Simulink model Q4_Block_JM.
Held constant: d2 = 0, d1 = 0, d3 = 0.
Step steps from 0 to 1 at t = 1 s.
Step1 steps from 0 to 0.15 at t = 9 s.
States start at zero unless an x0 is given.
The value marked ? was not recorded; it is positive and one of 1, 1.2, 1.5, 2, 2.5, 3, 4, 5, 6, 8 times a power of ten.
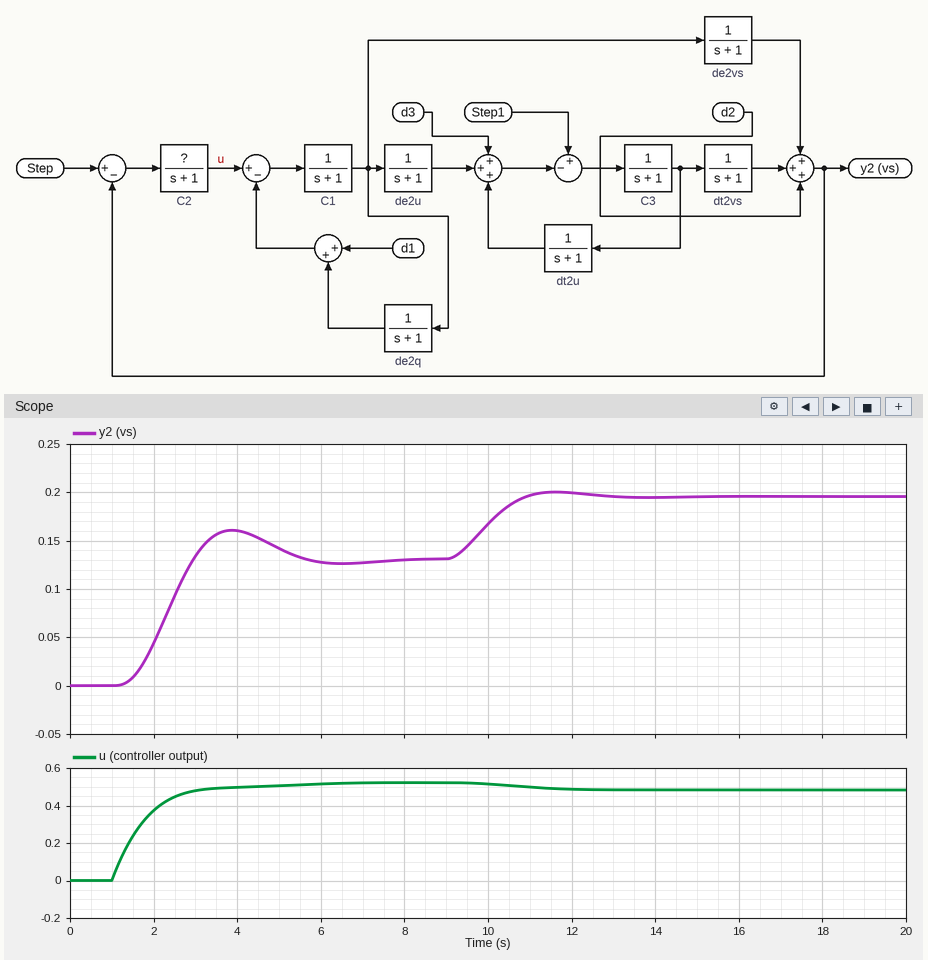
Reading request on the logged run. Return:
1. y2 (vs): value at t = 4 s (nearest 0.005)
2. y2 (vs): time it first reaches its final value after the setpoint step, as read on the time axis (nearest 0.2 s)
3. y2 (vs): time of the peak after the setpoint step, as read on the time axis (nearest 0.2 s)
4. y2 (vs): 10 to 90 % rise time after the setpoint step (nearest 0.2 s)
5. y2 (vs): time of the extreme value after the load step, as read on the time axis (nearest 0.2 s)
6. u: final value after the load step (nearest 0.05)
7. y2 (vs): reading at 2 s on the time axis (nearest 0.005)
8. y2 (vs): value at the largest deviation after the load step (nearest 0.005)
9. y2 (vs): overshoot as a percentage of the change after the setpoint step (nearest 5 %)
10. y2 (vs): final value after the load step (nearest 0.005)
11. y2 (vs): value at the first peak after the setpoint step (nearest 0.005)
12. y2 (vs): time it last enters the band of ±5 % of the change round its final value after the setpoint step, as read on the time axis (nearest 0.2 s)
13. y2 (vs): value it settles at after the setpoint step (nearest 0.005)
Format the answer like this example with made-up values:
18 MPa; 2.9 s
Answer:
0.160; 3.0 s; 3.8 s; 1.2 s; 11.6 s; 0.50; 0.045; 0.200; 25 %; 0.195; 0.160; 5.2 s; 0.130
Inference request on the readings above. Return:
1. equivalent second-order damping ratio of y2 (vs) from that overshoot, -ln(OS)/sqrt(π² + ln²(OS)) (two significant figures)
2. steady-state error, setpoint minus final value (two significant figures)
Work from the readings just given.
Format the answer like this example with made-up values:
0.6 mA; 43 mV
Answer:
0.40; 0.87
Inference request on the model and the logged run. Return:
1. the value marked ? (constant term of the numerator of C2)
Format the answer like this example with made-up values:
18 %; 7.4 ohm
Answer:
0.6
